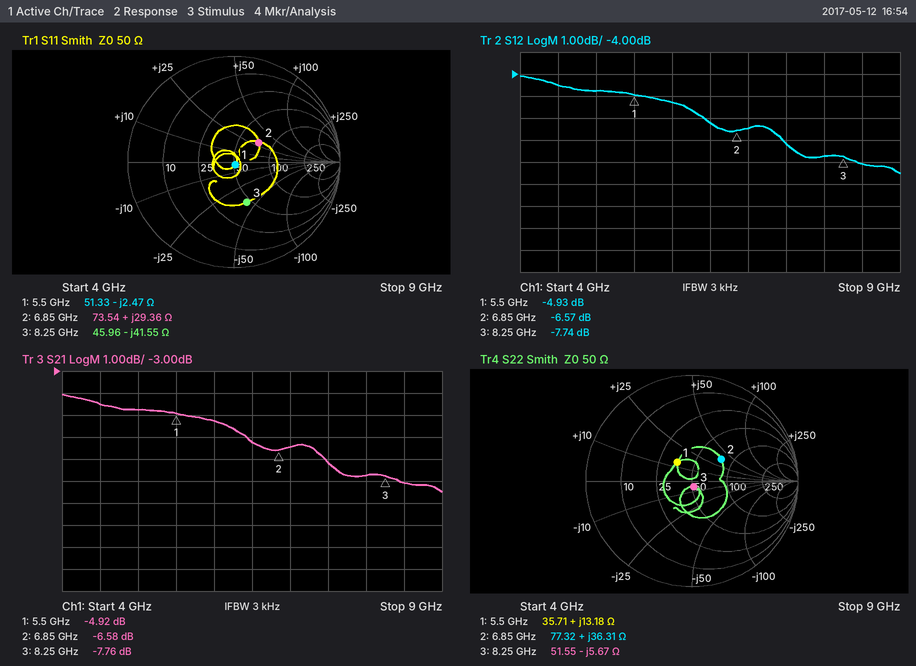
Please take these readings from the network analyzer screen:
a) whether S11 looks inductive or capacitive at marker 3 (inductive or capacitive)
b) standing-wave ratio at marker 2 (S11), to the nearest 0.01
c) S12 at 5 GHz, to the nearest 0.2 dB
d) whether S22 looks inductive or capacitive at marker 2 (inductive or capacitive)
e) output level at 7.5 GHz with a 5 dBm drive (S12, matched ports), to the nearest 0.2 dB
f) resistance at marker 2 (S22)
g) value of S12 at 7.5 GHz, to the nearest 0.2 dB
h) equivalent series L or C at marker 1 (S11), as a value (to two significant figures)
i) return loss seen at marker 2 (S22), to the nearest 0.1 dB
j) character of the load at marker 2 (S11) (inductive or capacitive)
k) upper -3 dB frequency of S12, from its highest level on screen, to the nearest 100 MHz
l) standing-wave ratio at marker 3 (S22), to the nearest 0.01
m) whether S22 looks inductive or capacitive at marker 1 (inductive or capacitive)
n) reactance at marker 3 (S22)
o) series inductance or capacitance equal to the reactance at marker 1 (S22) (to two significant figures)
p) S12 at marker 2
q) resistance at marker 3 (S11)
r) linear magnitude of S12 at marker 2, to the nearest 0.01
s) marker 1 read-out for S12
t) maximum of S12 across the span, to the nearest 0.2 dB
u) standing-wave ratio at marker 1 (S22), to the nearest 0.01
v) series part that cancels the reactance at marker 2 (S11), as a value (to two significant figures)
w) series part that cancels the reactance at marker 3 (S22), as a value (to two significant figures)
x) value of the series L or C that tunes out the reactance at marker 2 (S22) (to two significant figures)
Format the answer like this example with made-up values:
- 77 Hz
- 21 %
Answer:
- capacitive
- 1.84
- -4.8 dB
- inductive
- -2.2 dBm
- 77.32 Ω
- -7.2 dB
- 12 pF
- 9.3 dB
- inductive
- 7.5 GHz
- 1.12
- inductive
- -5.67 Ω
- 380 pH
- -6.57 dB
- 45.96 Ω
- 0.47
- -4.93 dB
- -4.0 dB
- 1.58
- 790 fF
- 110 pH
- 640 fF
